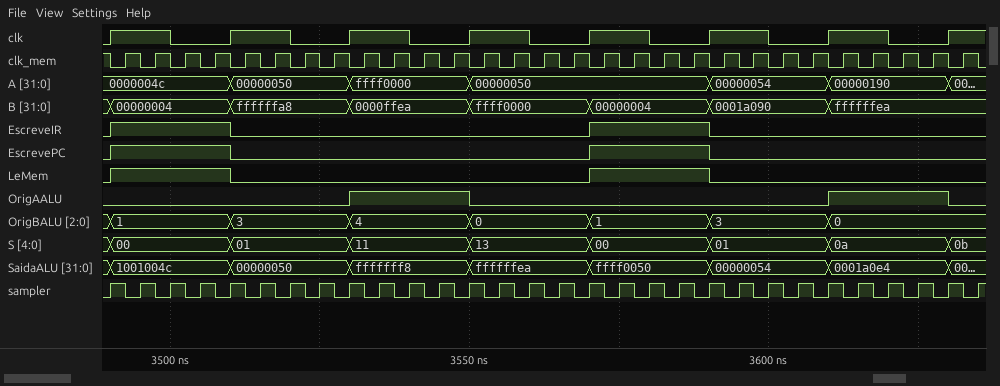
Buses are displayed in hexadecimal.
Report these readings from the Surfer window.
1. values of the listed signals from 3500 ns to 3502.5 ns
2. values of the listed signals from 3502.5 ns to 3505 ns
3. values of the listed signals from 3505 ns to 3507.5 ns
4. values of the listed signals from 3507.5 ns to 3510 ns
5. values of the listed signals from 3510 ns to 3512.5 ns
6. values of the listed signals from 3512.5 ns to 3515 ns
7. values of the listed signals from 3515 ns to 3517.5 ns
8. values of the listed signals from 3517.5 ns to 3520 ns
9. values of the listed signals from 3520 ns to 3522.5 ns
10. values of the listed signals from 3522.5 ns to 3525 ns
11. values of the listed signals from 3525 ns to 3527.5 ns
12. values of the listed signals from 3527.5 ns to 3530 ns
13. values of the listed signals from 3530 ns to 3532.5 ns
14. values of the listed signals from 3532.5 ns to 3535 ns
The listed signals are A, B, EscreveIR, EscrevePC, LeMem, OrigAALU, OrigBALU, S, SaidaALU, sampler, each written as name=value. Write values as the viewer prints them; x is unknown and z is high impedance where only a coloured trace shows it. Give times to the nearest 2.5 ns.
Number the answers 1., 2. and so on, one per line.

1. A=0000004c, B=00000004, EscreveIR=1, EscrevePC=1, LeMem=1, OrigAALU=0, OrigBALU=1, S=00, SaidaALU=1001004c, sampler=1
2. A=0000004c, B=00000004, EscreveIR=1, EscrevePC=1, LeMem=1, OrigAALU=0, OrigBALU=1, S=00, SaidaALU=1001004c, sampler=0
3. A=0000004c, B=00000004, EscreveIR=1, EscrevePC=1, LeMem=1, OrigAALU=0, OrigBALU=1, S=00, SaidaALU=1001004c, sampler=1
4. A=0000004c, B=00000004, EscreveIR=1, EscrevePC=1, LeMem=1, OrigAALU=0, OrigBALU=1, S=00, SaidaALU=1001004c, sampler=0
5. A=00000050, B=ffffffa8, EscreveIR=0, EscrevePC=0, LeMem=0, OrigAALU=0, OrigBALU=3, S=01, SaidaALU=00000050, sampler=1
6. A=00000050, B=ffffffa8, EscreveIR=0, EscrevePC=0, LeMem=0, OrigAALU=0, OrigBALU=3, S=01, SaidaALU=00000050, sampler=0
7. A=00000050, B=ffffffa8, EscreveIR=0, EscrevePC=0, LeMem=0, OrigAALU=0, OrigBALU=3, S=01, SaidaALU=00000050, sampler=1
8. A=00000050, B=ffffffa8, EscreveIR=0, EscrevePC=0, LeMem=0, OrigAALU=0, OrigBALU=3, S=01, SaidaALU=00000050, sampler=0
9. A=00000050, B=ffffffa8, EscreveIR=0, EscrevePC=0, LeMem=0, OrigAALU=0, OrigBALU=3, S=01, SaidaALU=00000050, sampler=1
10. A=00000050, B=ffffffa8, EscreveIR=0, EscrevePC=0, LeMem=0, OrigAALU=0, OrigBALU=3, S=01, SaidaALU=00000050, sampler=0
11. A=00000050, B=ffffffa8, EscreveIR=0, EscrevePC=0, LeMem=0, OrigAALU=0, OrigBALU=3, S=01, SaidaALU=00000050, sampler=1
12. A=00000050, B=ffffffa8, EscreveIR=0, EscrevePC=0, LeMem=0, OrigAALU=0, OrigBALU=3, S=01, SaidaALU=00000050, sampler=0
13. A=ffff0000, B=0000ffea, EscreveIR=0, EscrevePC=0, LeMem=0, OrigAALU=1, OrigBALU=4, S=11, SaidaALU=fffffff8, sampler=1
14. A=ffff0000, B=0000ffea, EscreveIR=0, EscrevePC=0, LeMem=0, OrigAALU=1, OrigBALU=4, S=11, SaidaALU=fffffff8, sampler=0
